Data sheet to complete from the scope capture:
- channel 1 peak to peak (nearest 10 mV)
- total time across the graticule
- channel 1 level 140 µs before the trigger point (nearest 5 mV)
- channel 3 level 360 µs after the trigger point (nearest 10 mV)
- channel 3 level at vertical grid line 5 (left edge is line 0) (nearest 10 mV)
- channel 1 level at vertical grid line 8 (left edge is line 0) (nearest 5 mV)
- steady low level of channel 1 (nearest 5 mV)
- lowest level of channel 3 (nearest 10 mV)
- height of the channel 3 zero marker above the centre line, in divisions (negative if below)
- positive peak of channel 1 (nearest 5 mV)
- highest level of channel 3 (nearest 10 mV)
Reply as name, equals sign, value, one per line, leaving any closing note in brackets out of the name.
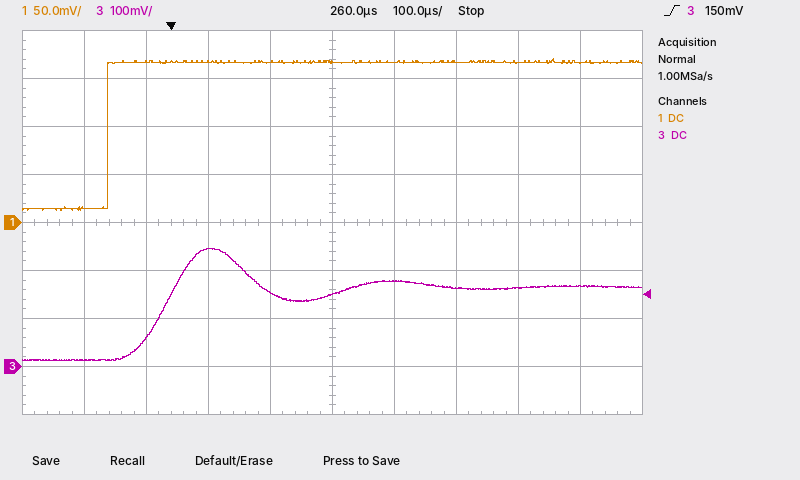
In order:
channel 1 peak to peak = 160 mV
total time across the graticule = 1 ms
channel 1 level 140 µs before the trigger point = 15 mV
channel 3 level 360 µs after the trigger point = 180 mV
channel 3 level at vertical grid line 5 (left edge is line 0) = 150 mV
channel 1 level at vertical grid line 8 (left edge is line 0) = 165 mV
steady low level of channel 1 = 15 mV
lowest level of channel 3 = 10 mV
height of the channel 3 zero marker above the centre line, in divisions = -3.0 div
positive peak of channel 1 = 170 mV
highest level of channel 3 = 250 mV
